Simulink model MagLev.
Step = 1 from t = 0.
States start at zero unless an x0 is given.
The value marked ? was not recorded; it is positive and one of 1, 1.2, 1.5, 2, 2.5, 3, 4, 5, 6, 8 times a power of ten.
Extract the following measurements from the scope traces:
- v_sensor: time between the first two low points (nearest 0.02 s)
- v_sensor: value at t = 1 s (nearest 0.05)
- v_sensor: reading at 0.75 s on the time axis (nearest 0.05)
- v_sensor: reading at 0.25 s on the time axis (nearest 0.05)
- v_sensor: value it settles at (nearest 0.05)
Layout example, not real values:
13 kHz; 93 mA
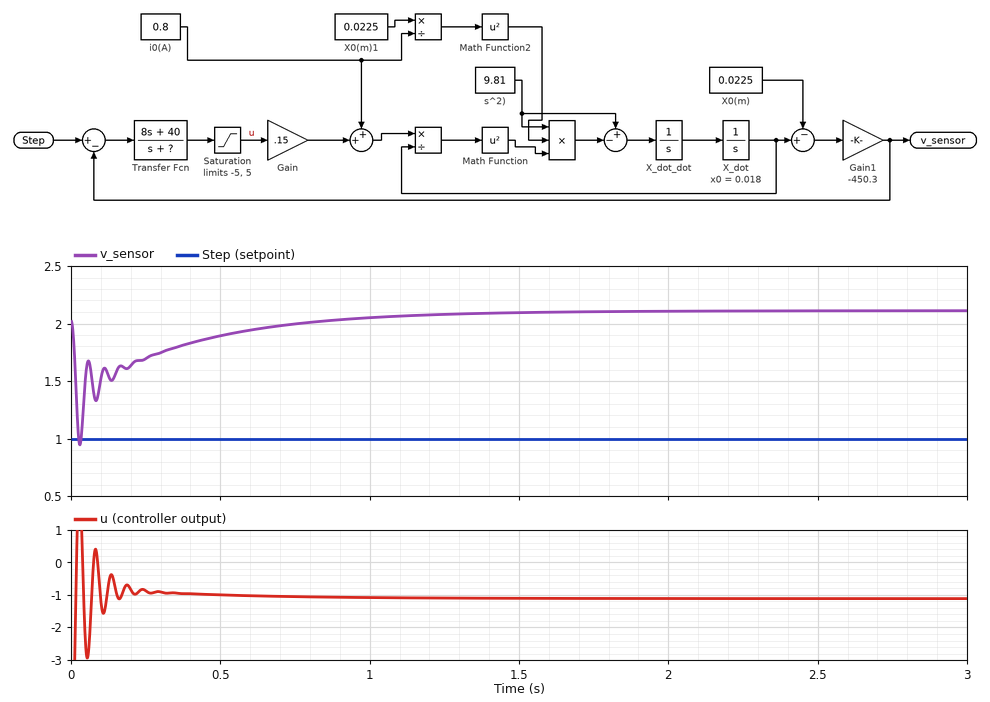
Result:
0.06 s; 2.05; 2.00; 1.70; 2.10
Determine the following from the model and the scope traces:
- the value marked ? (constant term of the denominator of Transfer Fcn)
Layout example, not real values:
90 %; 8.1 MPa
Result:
40
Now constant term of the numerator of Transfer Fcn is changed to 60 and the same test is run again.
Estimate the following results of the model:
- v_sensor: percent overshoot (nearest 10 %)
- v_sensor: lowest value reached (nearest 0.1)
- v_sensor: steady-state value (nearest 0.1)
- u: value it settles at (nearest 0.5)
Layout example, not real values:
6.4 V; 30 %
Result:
130 %; 0.9; 1.5; -1.0
